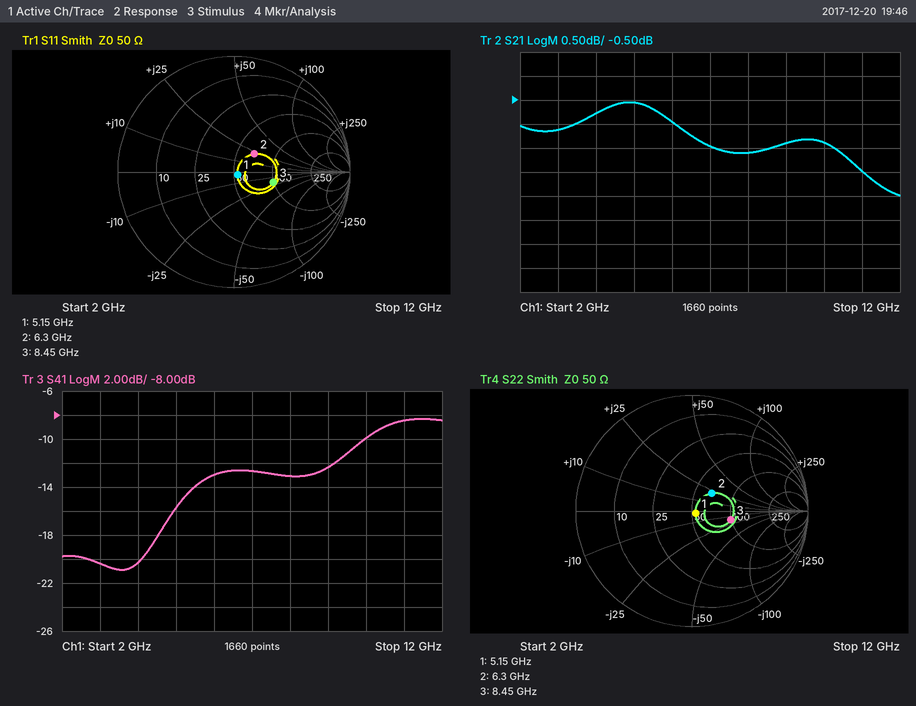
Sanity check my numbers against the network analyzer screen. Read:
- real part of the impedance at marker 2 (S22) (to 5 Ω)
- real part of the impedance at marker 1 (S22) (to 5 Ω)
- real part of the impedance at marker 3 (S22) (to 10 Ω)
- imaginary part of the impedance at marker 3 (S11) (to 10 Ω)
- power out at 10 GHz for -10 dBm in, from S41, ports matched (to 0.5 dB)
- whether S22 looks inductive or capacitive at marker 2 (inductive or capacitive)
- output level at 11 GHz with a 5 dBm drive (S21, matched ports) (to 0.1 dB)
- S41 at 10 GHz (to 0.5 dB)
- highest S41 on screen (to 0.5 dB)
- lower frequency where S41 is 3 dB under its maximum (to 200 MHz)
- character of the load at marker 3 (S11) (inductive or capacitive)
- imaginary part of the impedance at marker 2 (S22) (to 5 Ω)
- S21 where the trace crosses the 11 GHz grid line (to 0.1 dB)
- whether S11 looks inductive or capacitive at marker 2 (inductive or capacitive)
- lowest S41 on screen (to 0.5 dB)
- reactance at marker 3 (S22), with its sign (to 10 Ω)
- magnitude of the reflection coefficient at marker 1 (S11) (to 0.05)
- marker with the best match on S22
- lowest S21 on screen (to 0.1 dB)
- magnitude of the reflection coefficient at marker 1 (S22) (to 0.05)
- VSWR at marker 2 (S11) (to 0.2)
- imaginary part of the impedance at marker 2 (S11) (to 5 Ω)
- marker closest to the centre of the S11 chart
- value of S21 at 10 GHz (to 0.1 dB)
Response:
65 Ω
55 Ω
100 Ω
-20 Ω
-20.0 dBm
inductive
3.0 dBm
-10.0 dB
-8.5 dB
9.4 GHz
capacitive
+20 Ω
-2.0 dB
inductive
-21.0 dB
-20 Ω
0.05
marker 1
-2.5 dB
0.05
1.6
+20 Ω
marker 1
-1.4 dB
